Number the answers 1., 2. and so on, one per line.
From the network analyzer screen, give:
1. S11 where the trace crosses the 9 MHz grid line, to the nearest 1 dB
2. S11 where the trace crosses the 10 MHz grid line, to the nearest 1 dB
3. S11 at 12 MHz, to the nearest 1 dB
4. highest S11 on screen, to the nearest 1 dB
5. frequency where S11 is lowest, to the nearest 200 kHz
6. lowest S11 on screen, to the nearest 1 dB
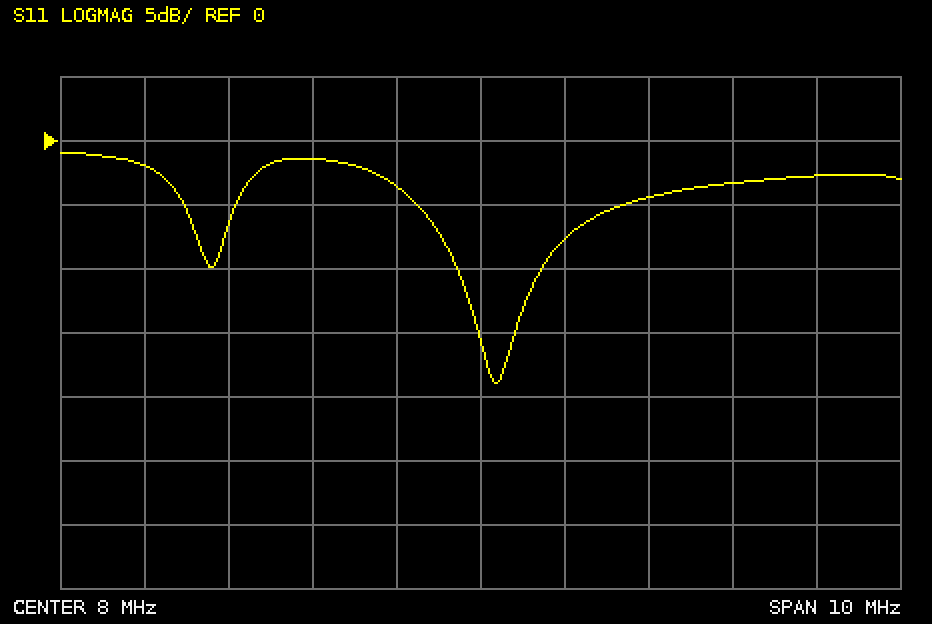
1. -8 dB
2. -4 dB
3. -3 dB
4. -1 dB
5. 8.2 MHz
6. -19 dB
